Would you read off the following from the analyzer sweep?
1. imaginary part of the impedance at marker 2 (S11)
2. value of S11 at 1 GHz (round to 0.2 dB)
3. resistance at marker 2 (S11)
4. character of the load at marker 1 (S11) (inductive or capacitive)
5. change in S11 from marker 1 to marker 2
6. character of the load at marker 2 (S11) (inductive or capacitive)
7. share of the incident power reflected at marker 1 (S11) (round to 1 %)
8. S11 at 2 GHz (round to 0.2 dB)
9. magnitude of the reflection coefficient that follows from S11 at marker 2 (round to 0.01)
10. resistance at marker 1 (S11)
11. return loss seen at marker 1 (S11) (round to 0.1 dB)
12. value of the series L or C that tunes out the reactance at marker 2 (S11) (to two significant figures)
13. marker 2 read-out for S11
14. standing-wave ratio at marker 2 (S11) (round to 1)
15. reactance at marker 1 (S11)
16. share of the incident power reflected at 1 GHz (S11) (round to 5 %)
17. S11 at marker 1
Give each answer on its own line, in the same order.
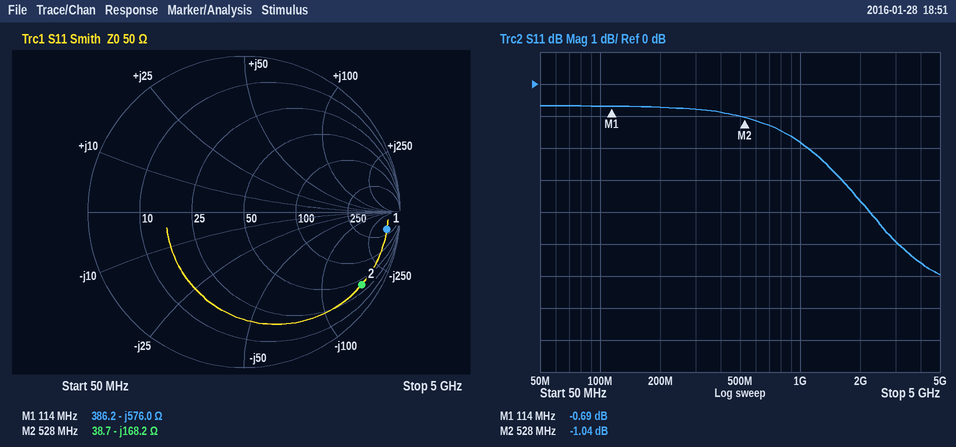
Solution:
-168.2 Ω
-1.8 dB
38.7 Ω
capacitive
-0.35 dB
capacitive
85 %
-3.6 dB
0.89
386.2 Ω
0.7 dB
51 nH
-1.04 dB
17
-576.0 Ω
65 %
-0.69 dB
